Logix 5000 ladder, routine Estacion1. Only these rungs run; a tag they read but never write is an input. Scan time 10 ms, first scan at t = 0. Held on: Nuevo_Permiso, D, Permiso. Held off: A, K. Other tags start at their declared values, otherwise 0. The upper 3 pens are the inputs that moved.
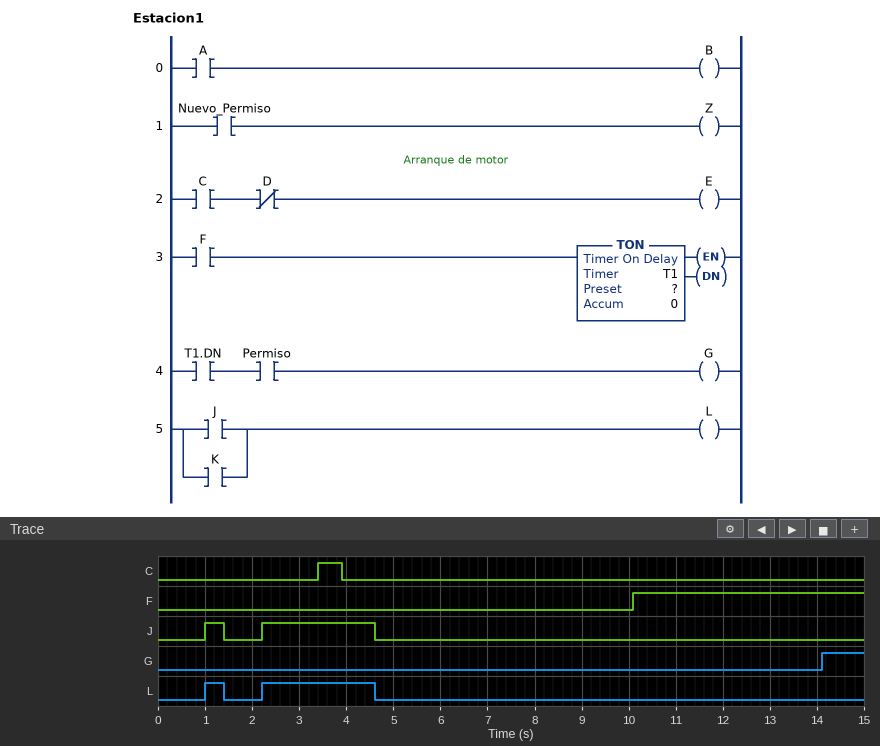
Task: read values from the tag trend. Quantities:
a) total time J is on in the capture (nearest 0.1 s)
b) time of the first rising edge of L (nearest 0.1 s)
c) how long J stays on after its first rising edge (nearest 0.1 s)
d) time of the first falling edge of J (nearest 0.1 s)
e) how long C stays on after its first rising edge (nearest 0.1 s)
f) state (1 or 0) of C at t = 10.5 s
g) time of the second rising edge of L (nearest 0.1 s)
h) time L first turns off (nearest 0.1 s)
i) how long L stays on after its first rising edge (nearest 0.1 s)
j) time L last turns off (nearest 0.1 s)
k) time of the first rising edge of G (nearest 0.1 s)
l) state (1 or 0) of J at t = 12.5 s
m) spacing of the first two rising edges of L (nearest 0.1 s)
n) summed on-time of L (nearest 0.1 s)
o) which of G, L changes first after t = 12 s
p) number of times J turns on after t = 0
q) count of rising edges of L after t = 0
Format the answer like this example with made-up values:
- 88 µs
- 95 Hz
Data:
- 2.8 s
- 1.0 s
- 0.4 s
- 1.4 s
- 0.5 s
- 0
- 2.2 s
- 1.4 s
- 0.4 s
- 4.6 s
- 14.1 s
- 0
- 1.2 s
- 2.8 s
- G
- 2
- 2
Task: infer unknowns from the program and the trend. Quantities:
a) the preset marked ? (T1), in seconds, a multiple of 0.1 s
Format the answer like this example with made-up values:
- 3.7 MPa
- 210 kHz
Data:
- 4.0 s
